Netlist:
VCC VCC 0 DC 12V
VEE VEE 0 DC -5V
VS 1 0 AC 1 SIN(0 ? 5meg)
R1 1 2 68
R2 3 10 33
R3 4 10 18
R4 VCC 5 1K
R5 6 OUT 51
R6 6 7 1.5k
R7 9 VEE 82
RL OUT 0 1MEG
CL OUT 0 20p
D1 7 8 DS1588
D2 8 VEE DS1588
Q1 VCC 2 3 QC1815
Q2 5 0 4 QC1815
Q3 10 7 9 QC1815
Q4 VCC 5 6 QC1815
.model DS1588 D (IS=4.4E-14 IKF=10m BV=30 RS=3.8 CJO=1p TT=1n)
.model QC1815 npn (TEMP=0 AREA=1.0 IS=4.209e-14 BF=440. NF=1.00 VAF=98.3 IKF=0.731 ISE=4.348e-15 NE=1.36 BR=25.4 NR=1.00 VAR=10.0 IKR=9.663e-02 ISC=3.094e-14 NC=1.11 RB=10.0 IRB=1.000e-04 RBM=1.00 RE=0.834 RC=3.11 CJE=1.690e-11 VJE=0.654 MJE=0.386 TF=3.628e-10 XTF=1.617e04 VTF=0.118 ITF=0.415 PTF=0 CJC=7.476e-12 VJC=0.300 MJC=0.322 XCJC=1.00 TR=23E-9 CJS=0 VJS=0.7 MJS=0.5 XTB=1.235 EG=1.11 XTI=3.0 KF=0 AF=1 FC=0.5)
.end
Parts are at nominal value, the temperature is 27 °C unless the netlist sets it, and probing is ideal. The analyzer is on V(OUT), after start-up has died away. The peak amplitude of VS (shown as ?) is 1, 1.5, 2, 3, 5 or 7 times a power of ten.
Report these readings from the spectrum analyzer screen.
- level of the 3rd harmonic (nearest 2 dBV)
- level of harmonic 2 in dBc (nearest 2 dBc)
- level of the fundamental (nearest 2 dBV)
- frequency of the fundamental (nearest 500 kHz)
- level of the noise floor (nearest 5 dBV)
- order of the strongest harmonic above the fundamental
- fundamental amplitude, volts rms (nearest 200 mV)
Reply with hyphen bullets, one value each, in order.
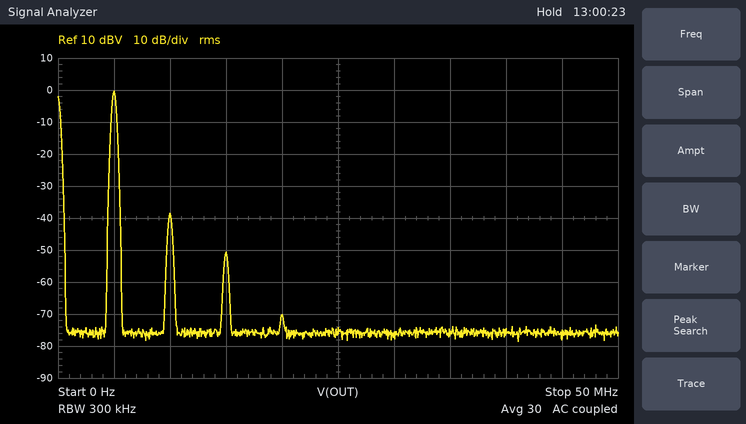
- -50 dBV
- -38 dBc
- 0 dBV
- 5.0 MHz
- -75 dBV
- 2
- 1.0 V
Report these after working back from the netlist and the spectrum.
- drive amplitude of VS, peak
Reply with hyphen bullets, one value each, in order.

- 100 mV
